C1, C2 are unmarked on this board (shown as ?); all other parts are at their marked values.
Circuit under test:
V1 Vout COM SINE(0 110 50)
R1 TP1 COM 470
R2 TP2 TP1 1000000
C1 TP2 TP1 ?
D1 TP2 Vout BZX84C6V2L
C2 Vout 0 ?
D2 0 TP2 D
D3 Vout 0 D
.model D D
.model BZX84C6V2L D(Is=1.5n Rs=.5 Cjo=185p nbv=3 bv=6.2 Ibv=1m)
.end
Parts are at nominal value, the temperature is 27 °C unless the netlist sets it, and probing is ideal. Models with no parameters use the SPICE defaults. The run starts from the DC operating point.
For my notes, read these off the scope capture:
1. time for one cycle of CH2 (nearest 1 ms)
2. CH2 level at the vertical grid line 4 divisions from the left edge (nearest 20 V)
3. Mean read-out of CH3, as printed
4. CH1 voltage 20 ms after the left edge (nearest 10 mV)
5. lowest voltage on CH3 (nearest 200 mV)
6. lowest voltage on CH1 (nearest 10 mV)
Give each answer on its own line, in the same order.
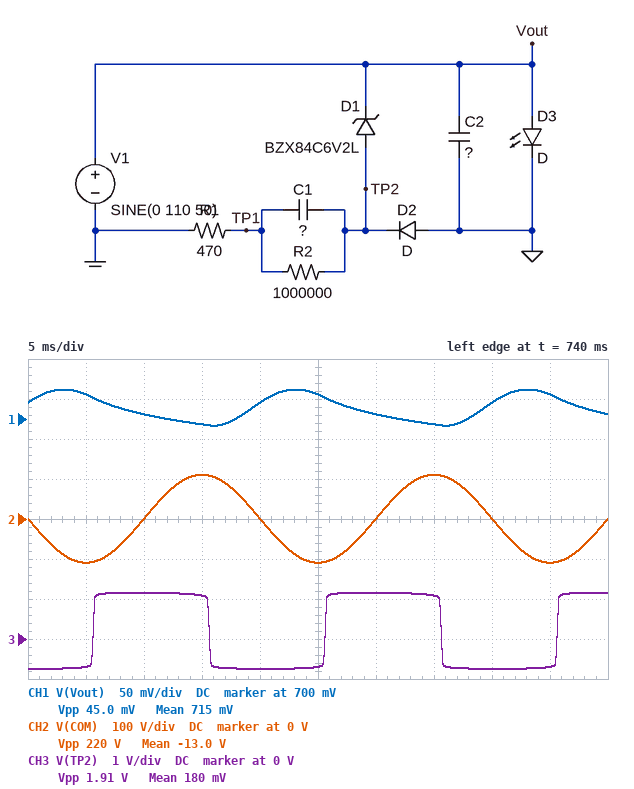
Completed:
20 ms
0 V
180 mV
720 mV
-800 mV
690 mV
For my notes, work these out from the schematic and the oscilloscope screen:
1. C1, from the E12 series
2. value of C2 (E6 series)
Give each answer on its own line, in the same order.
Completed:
1 µF
2.2 mF
